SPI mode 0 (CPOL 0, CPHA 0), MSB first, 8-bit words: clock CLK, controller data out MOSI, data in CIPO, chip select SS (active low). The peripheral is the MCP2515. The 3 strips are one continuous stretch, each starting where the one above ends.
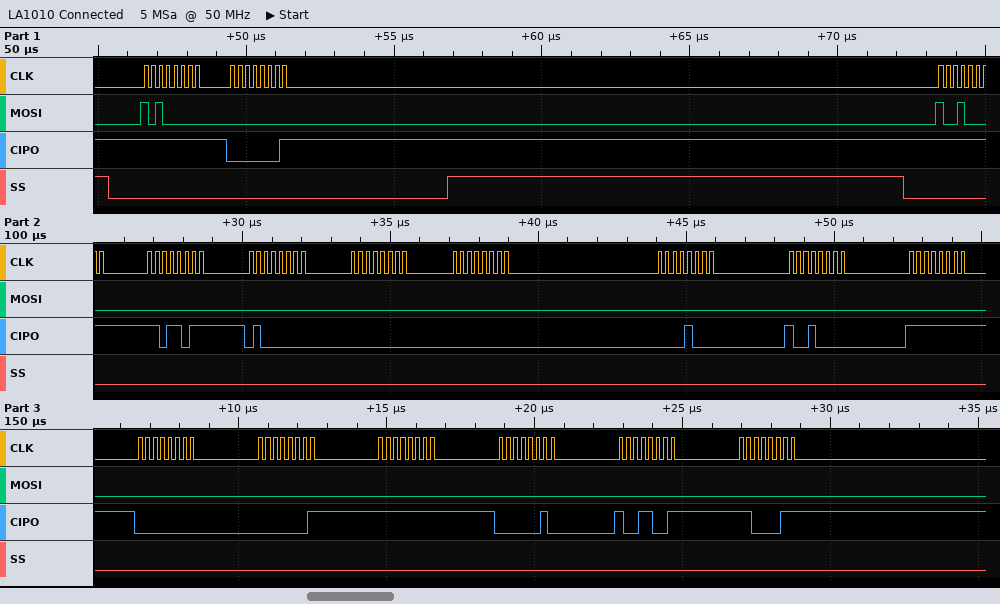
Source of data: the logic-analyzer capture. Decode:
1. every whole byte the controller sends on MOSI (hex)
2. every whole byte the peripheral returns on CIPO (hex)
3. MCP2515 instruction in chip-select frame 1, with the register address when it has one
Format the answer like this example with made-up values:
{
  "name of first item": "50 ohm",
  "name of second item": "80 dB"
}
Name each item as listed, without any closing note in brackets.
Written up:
{
  "every whole byte the controller sends on MOSI": "A0 00 90 00 00 00 00 00 00 00 00 00 00 00 00 00",
  "every whole byte the peripheral returns on CIPO": "FF 01 FF DB 40 00 00 08 90 FF 00 01 FF 02 99 C3",
  "MCP2515 instruction in chip-select frame 1, with the register address when it has one": "READ STATUS"
}
